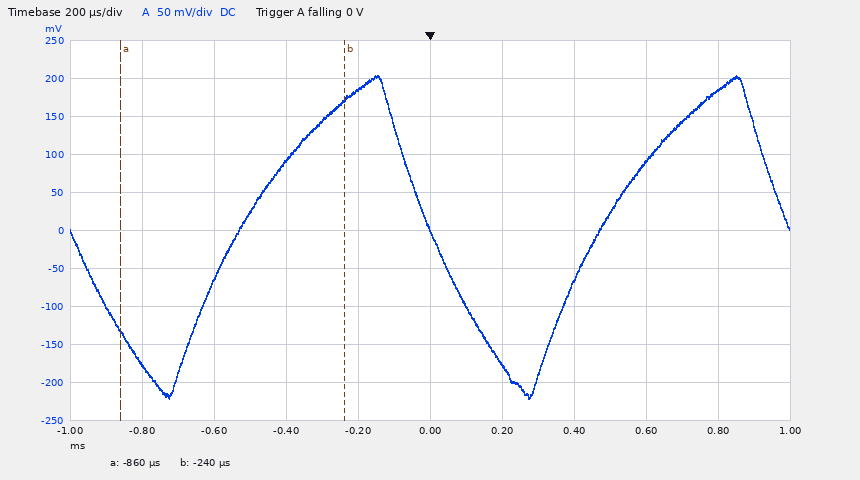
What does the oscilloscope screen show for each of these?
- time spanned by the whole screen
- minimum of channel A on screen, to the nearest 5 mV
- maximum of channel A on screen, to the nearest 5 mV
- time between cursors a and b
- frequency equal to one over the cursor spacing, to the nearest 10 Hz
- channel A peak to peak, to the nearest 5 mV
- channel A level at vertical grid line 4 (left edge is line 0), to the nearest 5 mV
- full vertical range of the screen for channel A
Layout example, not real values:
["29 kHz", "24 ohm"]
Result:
["2 ms", "-220 mV", "205 mV", "620 µs", "1.61 kHz", "425 mV", "185 mV", "500 mV"]
